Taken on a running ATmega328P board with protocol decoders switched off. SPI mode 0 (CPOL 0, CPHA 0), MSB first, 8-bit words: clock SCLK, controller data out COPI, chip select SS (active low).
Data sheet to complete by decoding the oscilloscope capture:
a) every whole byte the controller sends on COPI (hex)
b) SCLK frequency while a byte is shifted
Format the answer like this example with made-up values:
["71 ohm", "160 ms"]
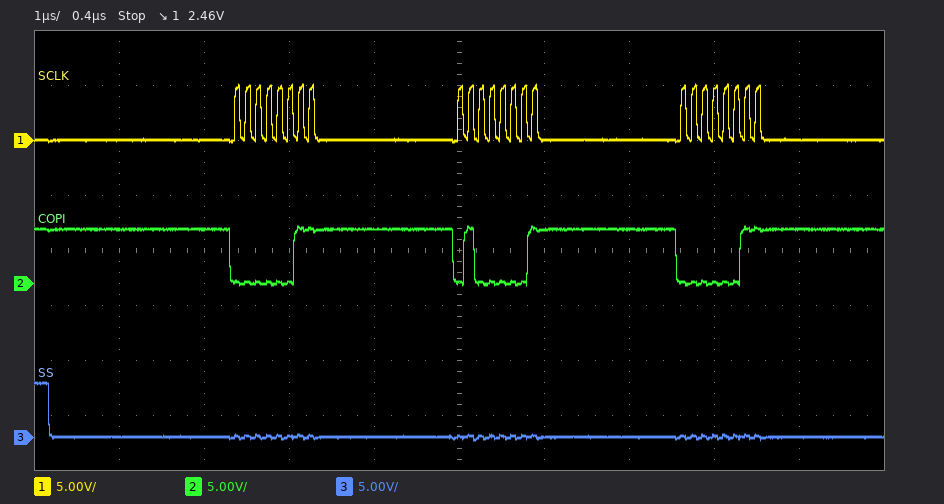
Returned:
["0x03 0x41 0x03", "8 MHz"]
